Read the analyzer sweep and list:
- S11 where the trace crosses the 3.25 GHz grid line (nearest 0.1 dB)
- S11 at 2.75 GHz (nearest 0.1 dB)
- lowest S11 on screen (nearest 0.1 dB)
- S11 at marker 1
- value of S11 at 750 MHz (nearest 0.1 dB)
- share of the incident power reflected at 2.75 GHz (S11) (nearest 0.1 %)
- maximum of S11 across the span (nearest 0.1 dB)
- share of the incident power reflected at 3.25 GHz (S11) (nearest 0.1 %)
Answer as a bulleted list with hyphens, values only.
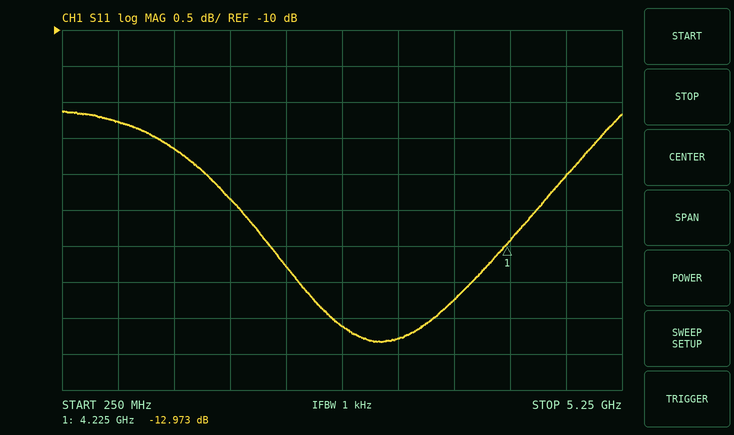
- -14.3 dB
- -14.1 dB
- -14.3 dB
- -12.973 dB
- -11.3 dB
- 3.9 %
- -11.1 dB
- 3.7 %
